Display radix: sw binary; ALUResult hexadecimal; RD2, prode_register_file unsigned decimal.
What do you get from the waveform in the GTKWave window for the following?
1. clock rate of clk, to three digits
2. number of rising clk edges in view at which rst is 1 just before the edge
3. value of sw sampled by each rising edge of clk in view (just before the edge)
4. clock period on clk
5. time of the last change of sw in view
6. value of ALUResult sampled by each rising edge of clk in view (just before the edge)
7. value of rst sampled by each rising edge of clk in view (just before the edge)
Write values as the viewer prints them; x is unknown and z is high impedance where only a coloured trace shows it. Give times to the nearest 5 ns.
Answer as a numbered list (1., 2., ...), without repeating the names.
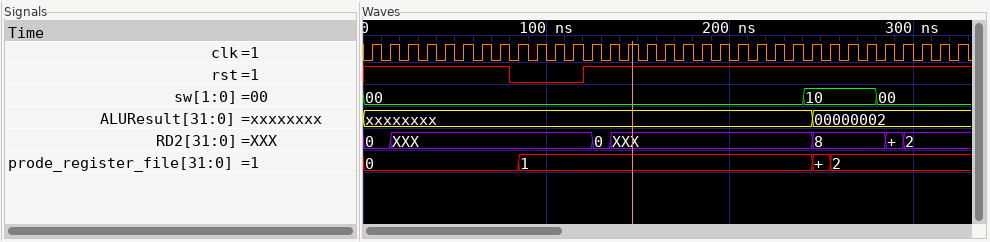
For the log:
1. 100 MHz
2. 29
3. 00, 00, 00, 00, 00, 00, 00, 00, 00, 00, 00, 00, 00, 00, 00, 00, 00, 00, 00, 00, 00, 00, 00, 00, 10, 10, 10, 10, 00, 00, 00, 00, 00
4. 10 ns
5. 280 ns
6. xxxxxxxx, xxxxxxxx, xxxxxxxx, xxxxxxxx, xxxxxxxx, xxxxxxxx, xxxxxxxx, xxxxxxxx, xxxxxxxx, xxxxxxxx, xxxxxxxx, xxxxxxxx, xxxxxxxx, xxxxxxxx, xxxxxxxx, xxxxxxxx, xxxxxxxx, xxxxxxxx, xxxxxxxx, xxxxxxxx, xxxxxxxx, xxxxxxxx, xxxxxxxx, xxxxxxxx, xxxxxxxx, 00000002, 00000002, 00000002, 00000002, 00000002, 00000002, 00000002, 00000002
7. 1 1 1 1 1 1 1 1 0 0 0 0 1 1 1 1 1 1 1 1 1 1 1 1 1 1 1 1 1 1 1 1 1
